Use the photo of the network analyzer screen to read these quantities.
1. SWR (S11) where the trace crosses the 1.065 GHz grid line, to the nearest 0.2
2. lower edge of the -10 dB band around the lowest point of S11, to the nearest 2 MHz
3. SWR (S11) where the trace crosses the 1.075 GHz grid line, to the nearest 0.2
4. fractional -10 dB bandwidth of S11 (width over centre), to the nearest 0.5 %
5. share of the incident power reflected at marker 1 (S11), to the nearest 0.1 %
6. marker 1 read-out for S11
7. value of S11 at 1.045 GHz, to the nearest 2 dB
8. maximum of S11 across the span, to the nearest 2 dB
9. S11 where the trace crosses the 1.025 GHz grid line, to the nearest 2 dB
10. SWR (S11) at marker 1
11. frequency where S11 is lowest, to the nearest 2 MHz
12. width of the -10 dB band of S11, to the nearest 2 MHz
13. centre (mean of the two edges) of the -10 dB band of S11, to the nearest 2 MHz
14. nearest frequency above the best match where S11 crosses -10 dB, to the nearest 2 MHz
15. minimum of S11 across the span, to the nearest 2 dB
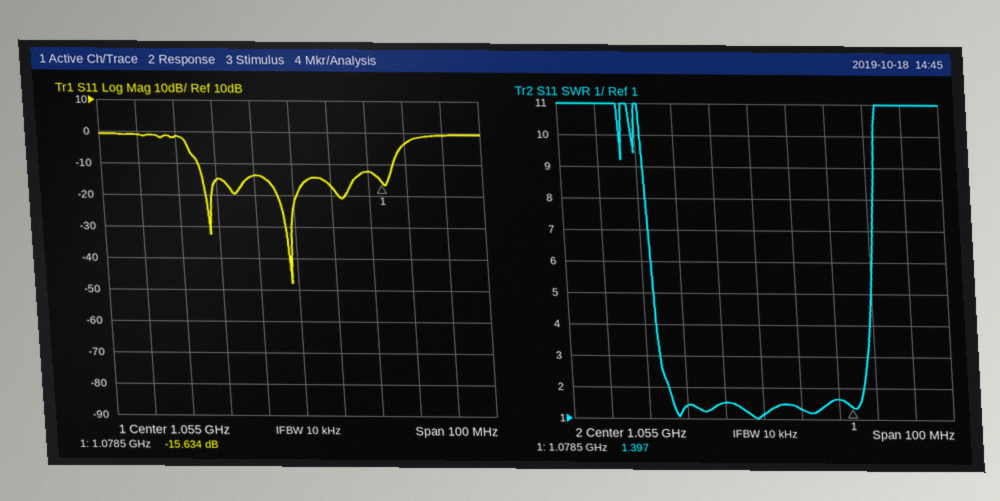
1.4
1.030 GHz
1.6
5.0 %
2.7 %
-15.634 dB
-14 dB
0 dB
-2 dB
1.397
1.054 GHz
52 MHz
1.056 GHz
1.082 GHz
-48 dB
